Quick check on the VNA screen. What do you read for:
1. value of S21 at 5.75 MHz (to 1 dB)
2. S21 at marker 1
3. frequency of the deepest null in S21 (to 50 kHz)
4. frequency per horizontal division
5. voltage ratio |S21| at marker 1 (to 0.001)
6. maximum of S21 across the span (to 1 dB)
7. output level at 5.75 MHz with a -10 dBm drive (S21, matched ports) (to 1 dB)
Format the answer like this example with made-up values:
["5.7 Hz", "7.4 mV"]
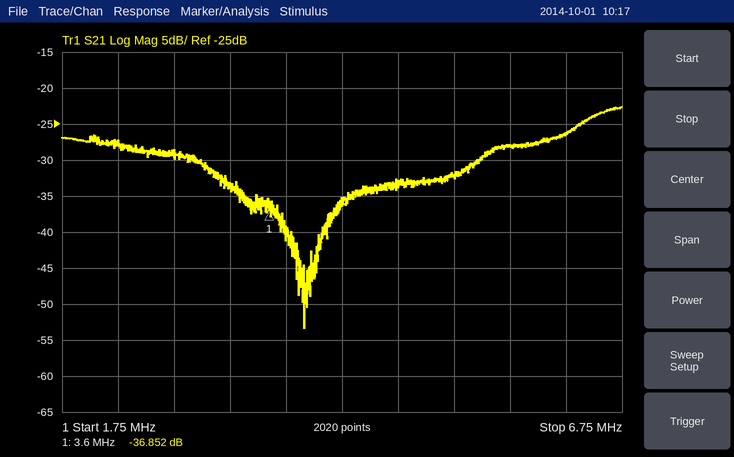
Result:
["-28 dB", "-36.852 dB", "3.90 MHz", "500 kHz", "0.014", "-23 dB", "-38 dBm"]
